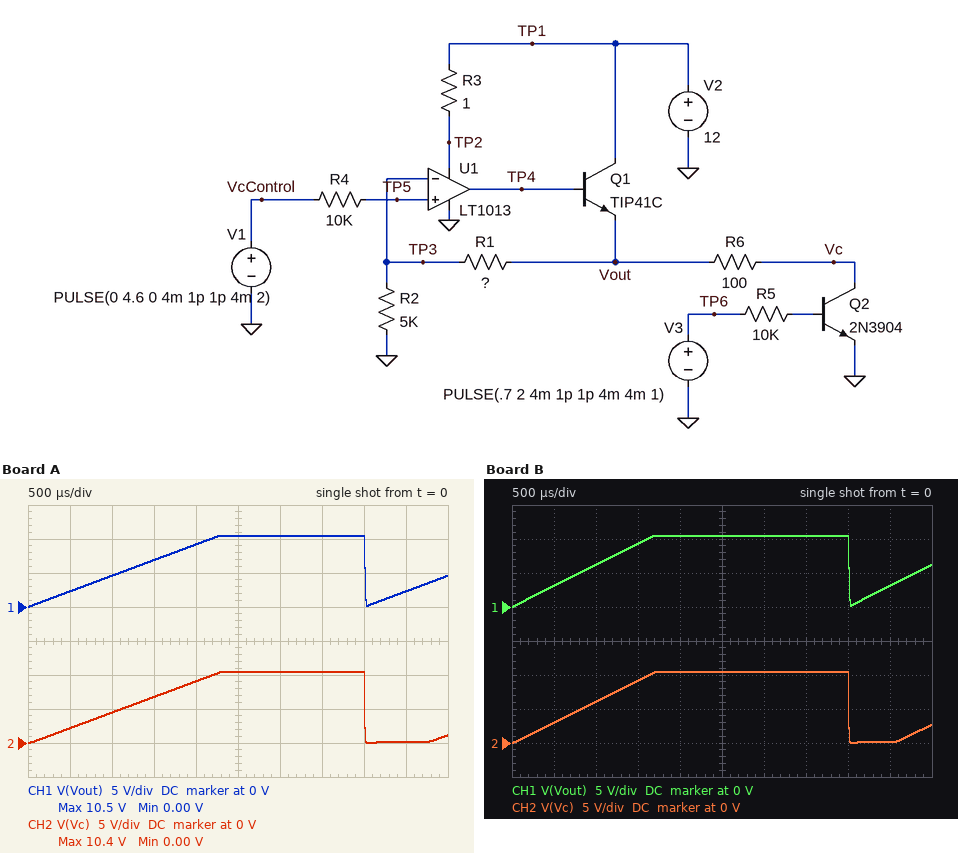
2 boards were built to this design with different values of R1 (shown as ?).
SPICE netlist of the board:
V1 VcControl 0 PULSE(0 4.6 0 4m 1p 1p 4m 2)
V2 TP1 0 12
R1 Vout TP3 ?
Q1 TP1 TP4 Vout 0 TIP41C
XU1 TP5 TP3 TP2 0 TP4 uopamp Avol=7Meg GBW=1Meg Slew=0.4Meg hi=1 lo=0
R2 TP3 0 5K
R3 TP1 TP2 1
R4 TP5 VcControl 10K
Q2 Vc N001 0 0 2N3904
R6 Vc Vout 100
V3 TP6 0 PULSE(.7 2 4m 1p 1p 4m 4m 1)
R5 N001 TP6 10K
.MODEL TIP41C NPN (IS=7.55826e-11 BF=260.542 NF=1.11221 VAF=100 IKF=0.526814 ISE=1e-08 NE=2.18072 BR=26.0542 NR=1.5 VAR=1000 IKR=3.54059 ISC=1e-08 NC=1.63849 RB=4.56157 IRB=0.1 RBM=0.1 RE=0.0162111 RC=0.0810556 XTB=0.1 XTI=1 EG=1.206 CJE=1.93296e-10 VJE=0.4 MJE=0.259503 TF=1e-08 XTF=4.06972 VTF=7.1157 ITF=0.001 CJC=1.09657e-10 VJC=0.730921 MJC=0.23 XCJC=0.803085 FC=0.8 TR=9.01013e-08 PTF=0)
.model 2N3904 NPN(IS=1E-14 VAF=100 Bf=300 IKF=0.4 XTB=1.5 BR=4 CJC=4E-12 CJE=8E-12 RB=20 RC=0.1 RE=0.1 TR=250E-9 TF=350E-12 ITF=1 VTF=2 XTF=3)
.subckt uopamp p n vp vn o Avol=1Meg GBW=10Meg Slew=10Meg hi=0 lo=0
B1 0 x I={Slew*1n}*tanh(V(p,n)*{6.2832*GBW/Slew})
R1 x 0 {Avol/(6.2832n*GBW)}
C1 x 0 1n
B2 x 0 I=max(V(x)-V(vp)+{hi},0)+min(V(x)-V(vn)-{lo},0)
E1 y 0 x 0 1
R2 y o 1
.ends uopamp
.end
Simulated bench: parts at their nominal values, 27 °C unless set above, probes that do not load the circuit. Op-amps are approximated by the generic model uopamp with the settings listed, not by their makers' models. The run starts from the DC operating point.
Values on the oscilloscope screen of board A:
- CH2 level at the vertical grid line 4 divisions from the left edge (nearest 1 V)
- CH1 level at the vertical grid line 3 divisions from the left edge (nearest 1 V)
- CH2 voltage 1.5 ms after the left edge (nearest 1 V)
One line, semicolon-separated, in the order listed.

9 V; 7 V; 7 V
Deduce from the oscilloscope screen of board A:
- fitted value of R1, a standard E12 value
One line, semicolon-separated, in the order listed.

15 kΩ
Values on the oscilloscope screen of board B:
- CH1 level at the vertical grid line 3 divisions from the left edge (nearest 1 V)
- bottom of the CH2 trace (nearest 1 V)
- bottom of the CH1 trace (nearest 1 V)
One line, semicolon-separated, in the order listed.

9 V; 0 V; 0 V
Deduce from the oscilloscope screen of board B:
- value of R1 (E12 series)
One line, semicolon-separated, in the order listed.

22 kΩ
